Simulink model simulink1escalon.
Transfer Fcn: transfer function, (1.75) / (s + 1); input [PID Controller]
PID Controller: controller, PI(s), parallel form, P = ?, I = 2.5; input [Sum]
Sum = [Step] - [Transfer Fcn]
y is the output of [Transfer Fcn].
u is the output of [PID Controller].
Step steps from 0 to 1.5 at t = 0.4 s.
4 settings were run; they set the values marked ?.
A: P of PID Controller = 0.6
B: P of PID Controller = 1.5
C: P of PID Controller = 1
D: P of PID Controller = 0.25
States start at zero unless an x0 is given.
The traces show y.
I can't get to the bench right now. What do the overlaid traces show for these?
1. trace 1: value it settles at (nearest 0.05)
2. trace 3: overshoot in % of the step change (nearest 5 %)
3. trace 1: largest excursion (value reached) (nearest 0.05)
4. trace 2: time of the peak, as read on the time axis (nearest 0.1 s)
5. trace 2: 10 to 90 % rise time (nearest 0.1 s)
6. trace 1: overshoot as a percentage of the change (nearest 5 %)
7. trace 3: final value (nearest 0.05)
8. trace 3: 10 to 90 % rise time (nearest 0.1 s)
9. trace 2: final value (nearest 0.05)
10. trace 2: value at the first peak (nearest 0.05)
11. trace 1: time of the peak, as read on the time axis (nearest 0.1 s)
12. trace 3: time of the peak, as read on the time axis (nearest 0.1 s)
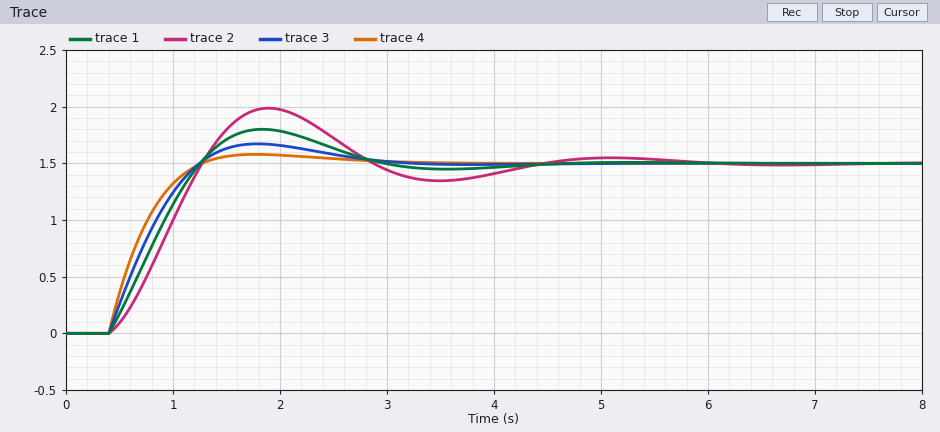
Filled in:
1.50
10 %
1.80
1.9 s
0.6 s
20 %
1.50
0.6 s
1.50
2.00
1.8 s
1.8 s
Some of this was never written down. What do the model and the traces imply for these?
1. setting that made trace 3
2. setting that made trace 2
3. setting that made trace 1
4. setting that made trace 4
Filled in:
C
D
A
B
